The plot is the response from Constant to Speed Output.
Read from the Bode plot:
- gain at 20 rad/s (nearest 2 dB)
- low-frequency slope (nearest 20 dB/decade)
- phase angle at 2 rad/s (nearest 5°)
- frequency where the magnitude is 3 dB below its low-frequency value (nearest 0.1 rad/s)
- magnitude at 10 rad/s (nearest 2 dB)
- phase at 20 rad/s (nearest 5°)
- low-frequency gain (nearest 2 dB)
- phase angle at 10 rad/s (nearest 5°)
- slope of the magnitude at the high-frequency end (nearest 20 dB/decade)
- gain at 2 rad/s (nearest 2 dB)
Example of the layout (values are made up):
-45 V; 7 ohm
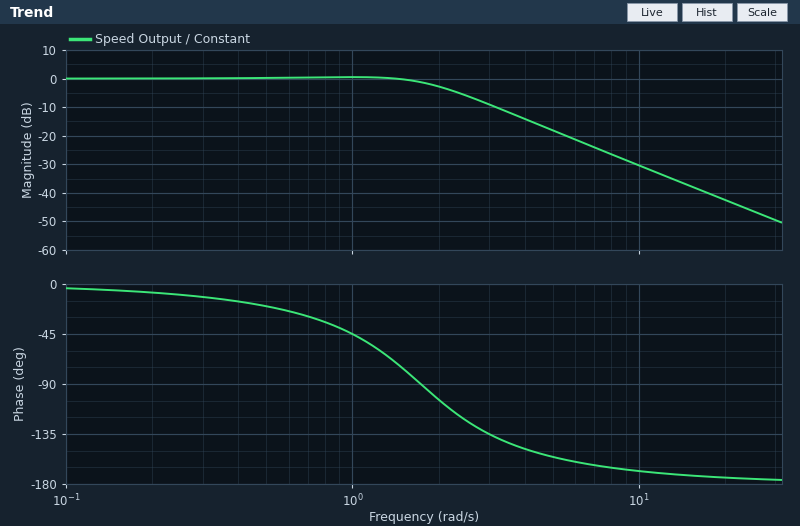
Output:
-42 dB; 0 dB/decade; -105°; 2.0 rad/s; -30 dB; -175°; 0 dB; -170°; -40 dB/decade; -2 dB
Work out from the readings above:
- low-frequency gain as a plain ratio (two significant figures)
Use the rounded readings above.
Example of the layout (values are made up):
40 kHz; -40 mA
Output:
1.0
